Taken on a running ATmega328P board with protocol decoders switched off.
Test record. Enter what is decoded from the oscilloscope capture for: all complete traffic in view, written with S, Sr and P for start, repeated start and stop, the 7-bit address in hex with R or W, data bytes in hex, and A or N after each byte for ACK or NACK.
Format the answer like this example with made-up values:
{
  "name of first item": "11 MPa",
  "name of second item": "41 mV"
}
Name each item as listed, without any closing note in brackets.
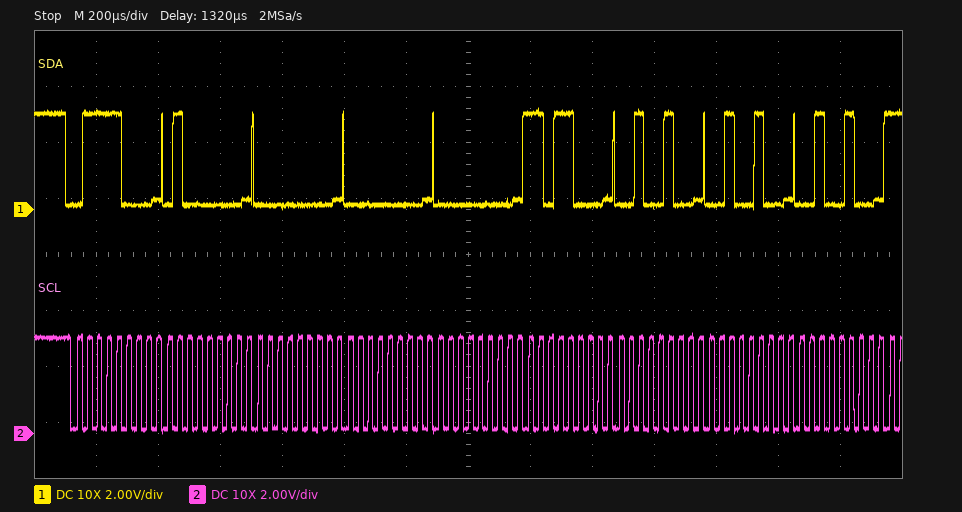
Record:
{
  "all complete traffic in view, written with S, Sr and P for start, repeated start and stop, the 7-bit address in hex with R or W, data bytes in hex, and A or N after each byte for ACK or NACK": "S 3CW A 40 A 00 A 00 A 00 A D8 A 24 A 24 A 24 A"
}
